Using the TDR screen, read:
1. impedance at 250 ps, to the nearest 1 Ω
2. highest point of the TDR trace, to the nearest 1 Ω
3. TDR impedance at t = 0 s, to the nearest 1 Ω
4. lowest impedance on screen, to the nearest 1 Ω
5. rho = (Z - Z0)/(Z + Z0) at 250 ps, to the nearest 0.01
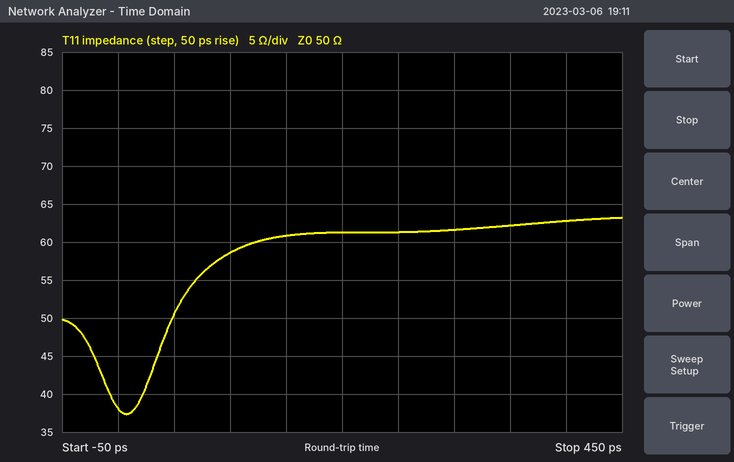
61 Ω
63 Ω
38 Ω
37 Ω
+0.10
